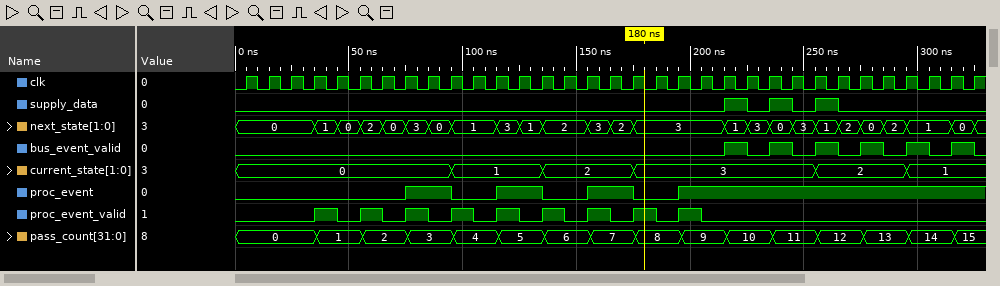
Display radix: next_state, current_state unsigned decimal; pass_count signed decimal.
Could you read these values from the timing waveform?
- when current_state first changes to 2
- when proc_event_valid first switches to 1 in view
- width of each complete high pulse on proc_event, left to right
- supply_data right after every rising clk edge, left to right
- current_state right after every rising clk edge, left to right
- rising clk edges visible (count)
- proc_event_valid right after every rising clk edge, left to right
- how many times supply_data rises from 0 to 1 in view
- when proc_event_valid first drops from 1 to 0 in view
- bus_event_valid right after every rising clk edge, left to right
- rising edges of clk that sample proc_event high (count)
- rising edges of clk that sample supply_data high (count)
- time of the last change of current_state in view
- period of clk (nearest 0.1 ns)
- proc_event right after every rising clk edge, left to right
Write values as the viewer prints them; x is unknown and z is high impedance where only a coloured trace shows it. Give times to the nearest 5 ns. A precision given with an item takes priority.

135 ns
35 ns
20 ns, 20 ns, 20 ns
0 0 0 0 0 0 0 0 0 0 0 0 0 0 0 0 0 0 0 0 0 1 0 1 0 1 0 0 0 0 0 0 0
0, 0, 0, 0, 0, 0, 0, 0, 0, 1, 1, 1, 1, 2, 2, 2, 2, 3, 3, 3, 3, 3, 3, 3, 3, 2, 2, 2, 2, 1, 1, 1, 1
33
0 0 0 1 0 1 0 1 0 1 0 1 0 1 0 1 0 1 0 1 0 0 0 0 0 0 0 0 0 0 0 0 0
3
45 ns
0 0 0 0 0 0 0 0 0 0 0 0 0 0 0 0 0 0 0 0 0 1 0 1 0 1 0 1 0 1 0 1 0
19
3
295 ns
10 ns
0 0 0 0 0 0 0 1 1 0 0 1 1 0 0 1 1 0 0 1 1 1 1 1 1 1 1 1 1 1 1 1 1
